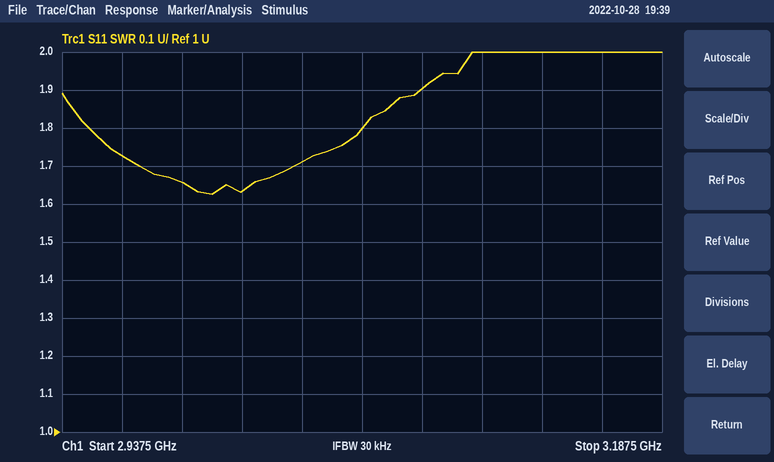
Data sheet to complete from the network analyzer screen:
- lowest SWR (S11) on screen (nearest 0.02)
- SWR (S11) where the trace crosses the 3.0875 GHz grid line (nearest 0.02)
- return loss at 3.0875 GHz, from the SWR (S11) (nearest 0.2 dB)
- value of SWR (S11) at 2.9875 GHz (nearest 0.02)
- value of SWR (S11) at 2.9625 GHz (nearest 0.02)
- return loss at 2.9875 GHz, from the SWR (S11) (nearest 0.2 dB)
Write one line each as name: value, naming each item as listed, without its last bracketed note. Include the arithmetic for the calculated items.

lowest SWR (S11) on screen: 1.62
SWR (S11) where the trace crosses the 3.0875 GHz grid line: 1.90
return loss at 3.0875 GHz, from the SWR (S11): −20 log10((1.9 − 1)/(1.9 + 1)) ≈ 10.2 dB
value of SWR (S11) at 2.9875 GHz: 1.66
value of SWR (S11) at 2.9625 GHz: 1.72
return loss at 2.9875 GHz, from the SWR (S11): −20 log10((1.66 − 1)/(1.66 + 1)) ≈ 12.1 dB, so 12.2 dB to the nearest 0.2 dB
